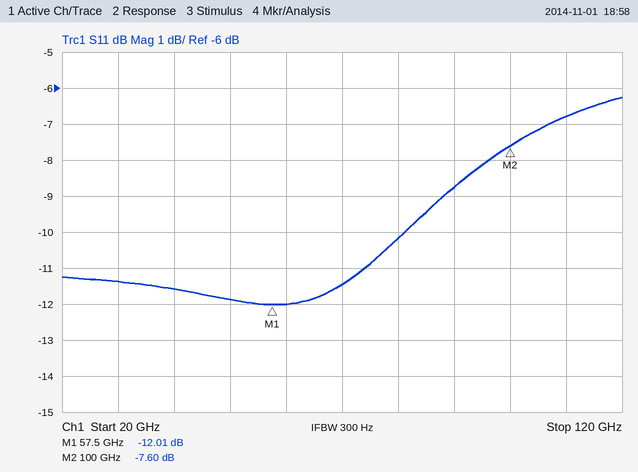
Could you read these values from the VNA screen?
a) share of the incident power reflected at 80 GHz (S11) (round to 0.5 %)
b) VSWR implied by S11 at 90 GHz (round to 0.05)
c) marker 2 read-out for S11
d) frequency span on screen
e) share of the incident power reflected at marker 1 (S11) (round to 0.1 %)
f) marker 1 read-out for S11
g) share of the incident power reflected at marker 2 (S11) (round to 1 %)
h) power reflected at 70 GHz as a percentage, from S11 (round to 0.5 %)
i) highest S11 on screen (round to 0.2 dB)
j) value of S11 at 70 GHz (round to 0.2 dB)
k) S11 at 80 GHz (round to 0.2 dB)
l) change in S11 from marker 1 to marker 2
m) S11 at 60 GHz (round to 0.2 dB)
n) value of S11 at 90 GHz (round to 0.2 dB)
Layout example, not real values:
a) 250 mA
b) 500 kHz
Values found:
a) 9.5 %
b) 2.15
c) -7.60 dB
d) 100 GHz
e) 6.3 %
f) -12.01 dB
g) 17 %
h) 7.0 %
i) -6.2 dB
j) -11.4 dB
k) -10.2 dB
l) 4.41 dB
m) -12.0 dB
n) -8.8 dB
